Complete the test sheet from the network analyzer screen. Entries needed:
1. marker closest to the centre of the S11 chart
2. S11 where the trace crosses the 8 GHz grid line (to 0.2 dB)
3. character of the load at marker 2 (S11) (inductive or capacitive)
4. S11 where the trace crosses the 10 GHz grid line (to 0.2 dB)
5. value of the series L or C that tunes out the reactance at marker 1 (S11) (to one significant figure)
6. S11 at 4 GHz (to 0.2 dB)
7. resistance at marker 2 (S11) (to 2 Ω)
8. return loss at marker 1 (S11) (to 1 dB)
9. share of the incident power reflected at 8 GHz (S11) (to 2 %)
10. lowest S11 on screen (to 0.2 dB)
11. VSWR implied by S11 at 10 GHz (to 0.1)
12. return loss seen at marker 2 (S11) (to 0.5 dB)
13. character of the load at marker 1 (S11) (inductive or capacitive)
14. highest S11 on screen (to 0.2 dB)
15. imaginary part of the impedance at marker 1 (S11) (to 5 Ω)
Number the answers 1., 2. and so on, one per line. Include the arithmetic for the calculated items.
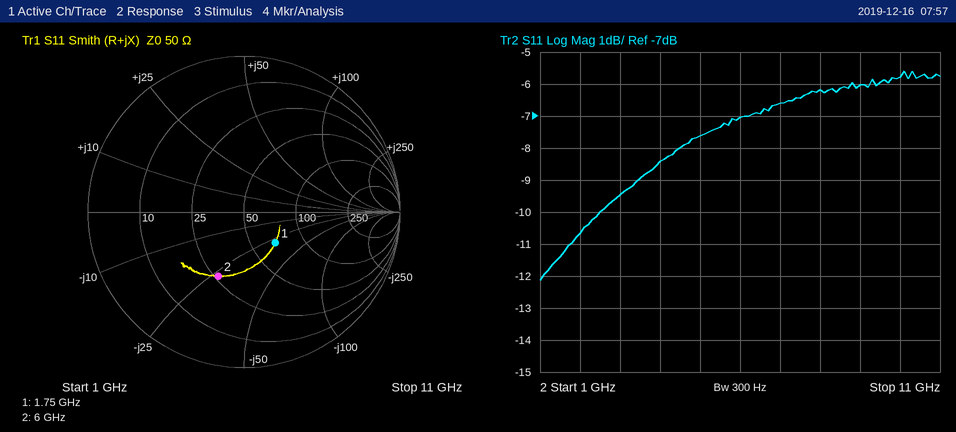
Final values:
1. marker 1
2. -6.2 dB
3. capacitive
4. -5.8 dB
5. L = 30 Ω/(2π × 1.75 GHz) ≈ 3 nH
6. -8.4 dB
7. 26 Ω
8. 11 dB
9. 10^(-6.2/10) ≈ 24 %
10. -12.2 dB
11. |Γ| = 10^(-5.8/20) = 0.5129; VSWR = (1 + 0.5129)/(1 − 0.5129) ≈ 3.1
12. 7.0 dB
13. capacitive
14. -5.6 dB
15. -30 Ω
